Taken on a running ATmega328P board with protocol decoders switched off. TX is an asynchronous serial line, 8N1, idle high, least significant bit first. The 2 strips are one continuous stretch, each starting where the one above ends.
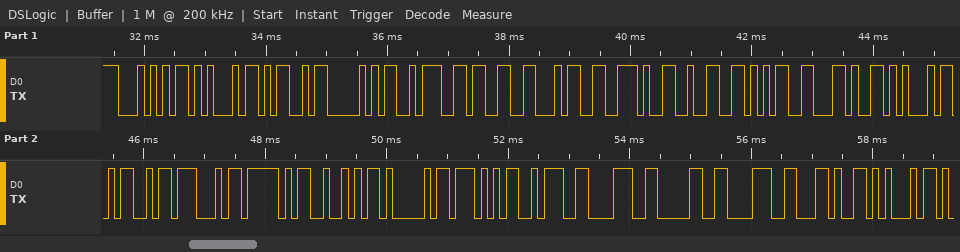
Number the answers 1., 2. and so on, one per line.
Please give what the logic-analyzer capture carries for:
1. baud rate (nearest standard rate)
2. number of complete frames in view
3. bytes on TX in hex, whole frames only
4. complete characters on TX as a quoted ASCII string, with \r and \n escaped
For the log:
1. 9600 baud
2. 24
3. 0x54 0x45 0x4D 0x50 0x3A 0x33 0x34 0x2E 0x32 0x35 0x2C 0x45 0x4D 0x47 0x5F 0x52 0x41 0x57 0x3A 0x38 0x30 0x38 0x2C 0x45
4. "TEMP:34.25,EMG_RAW:808,E"
